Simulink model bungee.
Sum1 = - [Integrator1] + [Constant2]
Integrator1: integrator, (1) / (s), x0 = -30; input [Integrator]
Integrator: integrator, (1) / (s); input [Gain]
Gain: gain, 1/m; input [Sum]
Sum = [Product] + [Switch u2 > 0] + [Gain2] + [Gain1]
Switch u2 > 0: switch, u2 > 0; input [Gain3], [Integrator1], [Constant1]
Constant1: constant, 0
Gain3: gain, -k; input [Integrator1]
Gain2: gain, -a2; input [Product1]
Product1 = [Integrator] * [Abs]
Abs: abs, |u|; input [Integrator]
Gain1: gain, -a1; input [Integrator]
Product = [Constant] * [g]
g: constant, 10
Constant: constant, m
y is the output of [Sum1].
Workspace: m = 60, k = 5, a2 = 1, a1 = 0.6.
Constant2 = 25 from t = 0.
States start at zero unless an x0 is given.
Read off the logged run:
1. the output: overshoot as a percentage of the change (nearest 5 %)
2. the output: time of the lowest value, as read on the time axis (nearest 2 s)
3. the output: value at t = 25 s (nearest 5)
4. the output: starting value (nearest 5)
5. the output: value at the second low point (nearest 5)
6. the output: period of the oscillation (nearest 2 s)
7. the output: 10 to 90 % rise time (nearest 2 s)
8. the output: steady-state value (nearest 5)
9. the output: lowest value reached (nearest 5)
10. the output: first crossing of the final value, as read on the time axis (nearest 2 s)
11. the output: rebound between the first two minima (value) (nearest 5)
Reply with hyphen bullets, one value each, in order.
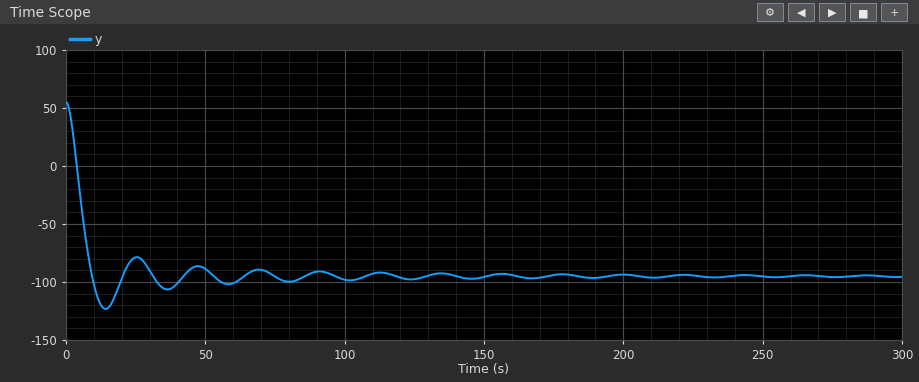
- 20 %
- 14 s
- -80
- 55
- -105
- 22 s
- 6 s
- -95
- -125
- 10 s
- -80
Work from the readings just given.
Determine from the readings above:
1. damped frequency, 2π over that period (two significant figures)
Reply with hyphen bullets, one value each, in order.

- 0.29 rad/s
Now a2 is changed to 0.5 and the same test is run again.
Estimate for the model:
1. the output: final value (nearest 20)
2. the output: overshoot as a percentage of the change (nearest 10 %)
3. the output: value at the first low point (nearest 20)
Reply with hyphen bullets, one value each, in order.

- -100
- 30 %
- -140
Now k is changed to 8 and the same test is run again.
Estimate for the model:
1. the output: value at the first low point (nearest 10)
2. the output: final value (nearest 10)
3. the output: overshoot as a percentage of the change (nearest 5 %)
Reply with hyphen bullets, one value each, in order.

- -80
- -50
- 25 %
